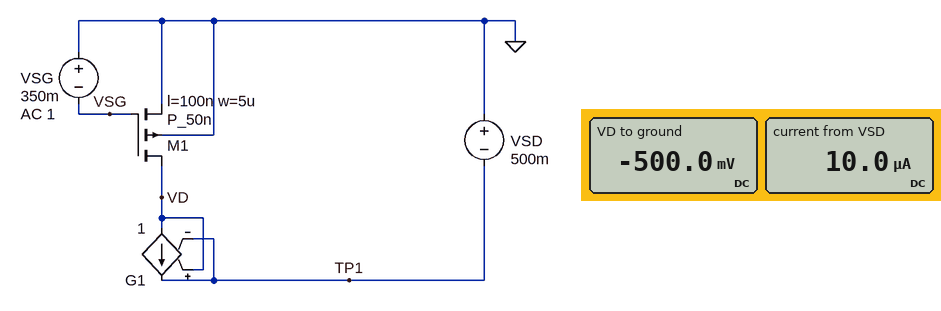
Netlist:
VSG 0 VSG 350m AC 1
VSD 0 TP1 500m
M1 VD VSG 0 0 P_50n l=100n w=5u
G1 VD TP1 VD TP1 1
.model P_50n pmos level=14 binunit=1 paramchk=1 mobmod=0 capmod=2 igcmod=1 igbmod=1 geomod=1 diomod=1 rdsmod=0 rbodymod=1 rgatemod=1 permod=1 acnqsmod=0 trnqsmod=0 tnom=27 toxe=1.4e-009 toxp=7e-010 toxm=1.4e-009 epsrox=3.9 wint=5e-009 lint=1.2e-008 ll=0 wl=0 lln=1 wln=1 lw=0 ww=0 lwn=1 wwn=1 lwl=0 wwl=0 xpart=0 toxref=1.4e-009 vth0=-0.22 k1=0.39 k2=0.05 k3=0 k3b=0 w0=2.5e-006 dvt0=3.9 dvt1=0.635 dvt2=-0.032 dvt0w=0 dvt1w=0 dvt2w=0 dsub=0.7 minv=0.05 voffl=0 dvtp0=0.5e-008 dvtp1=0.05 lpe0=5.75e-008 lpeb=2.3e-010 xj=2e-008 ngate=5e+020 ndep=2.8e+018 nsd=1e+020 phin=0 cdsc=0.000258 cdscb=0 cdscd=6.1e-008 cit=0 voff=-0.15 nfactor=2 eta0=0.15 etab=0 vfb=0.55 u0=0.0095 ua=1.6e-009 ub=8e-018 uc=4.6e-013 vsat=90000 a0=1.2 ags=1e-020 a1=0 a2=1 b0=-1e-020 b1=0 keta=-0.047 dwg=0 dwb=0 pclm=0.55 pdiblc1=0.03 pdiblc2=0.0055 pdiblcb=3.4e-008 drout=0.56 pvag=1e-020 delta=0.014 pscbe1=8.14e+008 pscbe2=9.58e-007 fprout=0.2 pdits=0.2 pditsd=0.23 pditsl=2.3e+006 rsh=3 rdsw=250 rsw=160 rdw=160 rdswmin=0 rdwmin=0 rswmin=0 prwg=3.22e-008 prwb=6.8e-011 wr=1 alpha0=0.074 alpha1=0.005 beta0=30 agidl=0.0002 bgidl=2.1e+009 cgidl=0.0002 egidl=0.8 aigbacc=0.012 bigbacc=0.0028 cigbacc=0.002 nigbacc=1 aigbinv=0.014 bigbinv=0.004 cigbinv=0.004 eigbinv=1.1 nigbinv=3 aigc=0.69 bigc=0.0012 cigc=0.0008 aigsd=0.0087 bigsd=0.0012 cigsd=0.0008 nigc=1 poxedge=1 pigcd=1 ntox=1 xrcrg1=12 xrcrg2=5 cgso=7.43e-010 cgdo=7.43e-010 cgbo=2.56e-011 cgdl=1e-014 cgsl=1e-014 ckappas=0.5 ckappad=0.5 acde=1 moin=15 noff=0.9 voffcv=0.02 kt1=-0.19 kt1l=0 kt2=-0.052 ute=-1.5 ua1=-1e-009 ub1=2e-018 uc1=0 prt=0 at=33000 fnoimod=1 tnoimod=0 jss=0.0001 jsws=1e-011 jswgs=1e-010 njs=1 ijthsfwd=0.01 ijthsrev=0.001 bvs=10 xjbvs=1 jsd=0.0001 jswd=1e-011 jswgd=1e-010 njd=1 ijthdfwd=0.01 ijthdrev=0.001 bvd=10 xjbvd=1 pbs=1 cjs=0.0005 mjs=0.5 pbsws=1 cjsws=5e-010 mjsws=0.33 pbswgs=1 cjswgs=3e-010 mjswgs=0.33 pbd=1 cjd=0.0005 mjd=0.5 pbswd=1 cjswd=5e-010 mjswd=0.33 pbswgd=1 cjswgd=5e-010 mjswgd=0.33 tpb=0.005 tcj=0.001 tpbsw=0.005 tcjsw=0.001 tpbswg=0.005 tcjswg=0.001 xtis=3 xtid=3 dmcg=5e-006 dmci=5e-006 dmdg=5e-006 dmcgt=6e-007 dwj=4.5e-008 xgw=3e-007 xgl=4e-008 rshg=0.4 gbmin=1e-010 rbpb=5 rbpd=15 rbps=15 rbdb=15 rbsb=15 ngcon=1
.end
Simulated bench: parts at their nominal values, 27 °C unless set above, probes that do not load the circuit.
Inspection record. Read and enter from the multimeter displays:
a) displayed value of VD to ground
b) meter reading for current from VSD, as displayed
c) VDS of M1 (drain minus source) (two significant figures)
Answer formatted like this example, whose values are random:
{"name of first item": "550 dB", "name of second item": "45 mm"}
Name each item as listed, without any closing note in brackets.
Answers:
{"displayed value of VD to ground": "-500.0 mV", "meter reading for current from VSD, as displayed": "10.0 µA", "VDS of M1 (drain minus source)": "-500 mV"}
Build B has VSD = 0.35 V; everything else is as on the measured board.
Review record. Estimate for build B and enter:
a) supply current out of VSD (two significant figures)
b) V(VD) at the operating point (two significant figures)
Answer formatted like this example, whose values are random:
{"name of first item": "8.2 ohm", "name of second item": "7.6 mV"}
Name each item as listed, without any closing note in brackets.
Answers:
{"supply current out of VSD": "9.5 µA", "V(VD) at the operating point": "-350 mV"}
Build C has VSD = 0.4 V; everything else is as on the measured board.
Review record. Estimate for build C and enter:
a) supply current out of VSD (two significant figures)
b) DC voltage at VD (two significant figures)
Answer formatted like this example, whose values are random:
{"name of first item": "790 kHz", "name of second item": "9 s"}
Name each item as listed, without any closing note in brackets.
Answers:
{"supply current out of VSD": "9.7 µA", "DC voltage at VD": "-400 mV"}
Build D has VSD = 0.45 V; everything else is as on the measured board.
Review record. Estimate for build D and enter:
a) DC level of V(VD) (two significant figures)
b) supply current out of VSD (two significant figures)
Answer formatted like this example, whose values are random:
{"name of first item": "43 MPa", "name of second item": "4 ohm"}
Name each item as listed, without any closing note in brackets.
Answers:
{"DC level of V(VD)": "-450 mV", "supply current out of VSD": "9.8 µA"}
